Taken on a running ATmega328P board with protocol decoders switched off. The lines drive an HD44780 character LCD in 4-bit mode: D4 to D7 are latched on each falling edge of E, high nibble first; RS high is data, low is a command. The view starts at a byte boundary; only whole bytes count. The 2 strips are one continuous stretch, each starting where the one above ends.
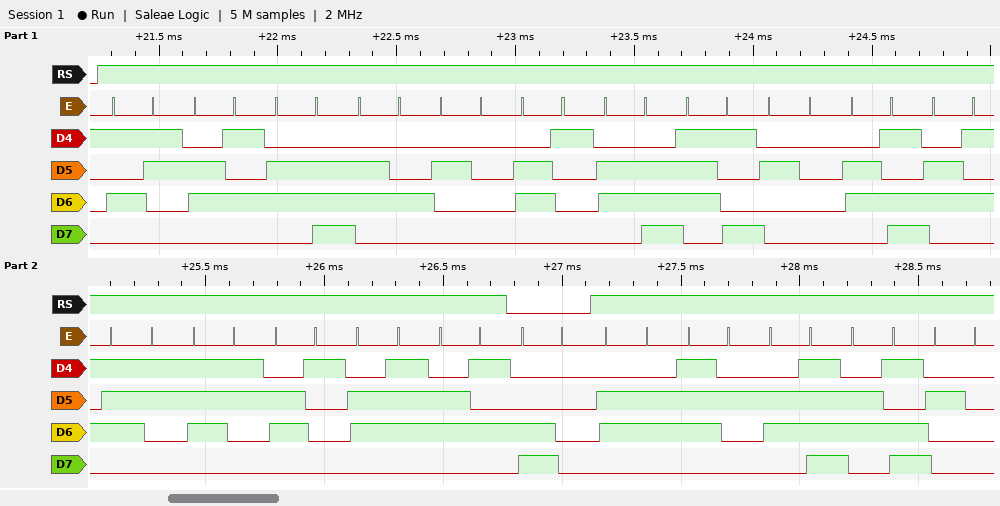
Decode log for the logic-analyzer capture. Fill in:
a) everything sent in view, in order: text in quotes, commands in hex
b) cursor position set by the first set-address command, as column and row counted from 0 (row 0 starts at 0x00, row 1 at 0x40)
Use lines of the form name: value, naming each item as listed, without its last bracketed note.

everything sent in view, in order: text in quotes, commands in hex: "Send any message" 0xC0 "from "
cursor position set by the first set-address command, as column and row counted from 0: column 0, row 1
